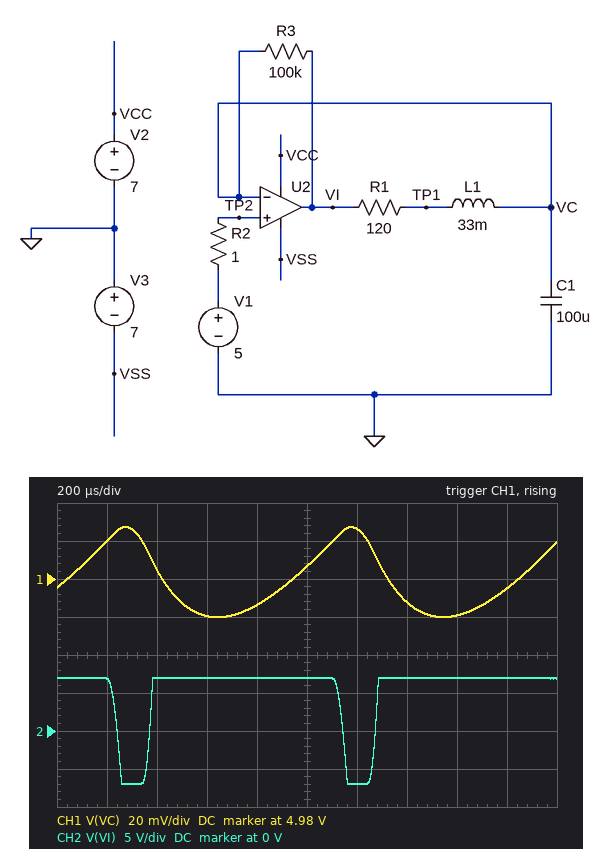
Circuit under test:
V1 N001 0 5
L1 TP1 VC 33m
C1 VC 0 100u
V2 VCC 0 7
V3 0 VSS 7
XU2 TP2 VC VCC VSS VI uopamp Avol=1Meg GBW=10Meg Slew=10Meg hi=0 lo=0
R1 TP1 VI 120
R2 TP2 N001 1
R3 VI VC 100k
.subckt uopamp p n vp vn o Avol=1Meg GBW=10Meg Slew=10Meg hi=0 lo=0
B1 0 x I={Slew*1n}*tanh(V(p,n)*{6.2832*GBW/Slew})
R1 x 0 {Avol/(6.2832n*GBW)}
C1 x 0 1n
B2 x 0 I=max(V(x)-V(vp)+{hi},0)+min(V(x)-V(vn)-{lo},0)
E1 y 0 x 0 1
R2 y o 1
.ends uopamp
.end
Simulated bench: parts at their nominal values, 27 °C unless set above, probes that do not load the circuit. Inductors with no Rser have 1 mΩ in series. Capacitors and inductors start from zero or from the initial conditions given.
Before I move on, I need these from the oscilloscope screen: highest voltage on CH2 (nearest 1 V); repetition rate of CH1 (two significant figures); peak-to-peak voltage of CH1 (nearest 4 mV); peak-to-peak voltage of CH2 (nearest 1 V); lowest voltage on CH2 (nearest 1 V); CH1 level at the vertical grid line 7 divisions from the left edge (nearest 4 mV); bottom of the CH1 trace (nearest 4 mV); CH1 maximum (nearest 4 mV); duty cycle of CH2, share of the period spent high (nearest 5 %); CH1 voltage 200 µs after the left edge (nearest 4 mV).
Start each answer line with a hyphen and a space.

- 7 V
- 1.1 kHz
- 48 mV
- 14 V
- -7 V
- 4.968 V
- 4.960 V
- 5.008 V
- 85 %
- 5.000 V
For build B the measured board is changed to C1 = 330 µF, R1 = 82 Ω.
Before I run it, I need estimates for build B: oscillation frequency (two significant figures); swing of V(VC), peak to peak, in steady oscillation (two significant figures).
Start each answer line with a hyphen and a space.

- 740 Hz
- 32 mV
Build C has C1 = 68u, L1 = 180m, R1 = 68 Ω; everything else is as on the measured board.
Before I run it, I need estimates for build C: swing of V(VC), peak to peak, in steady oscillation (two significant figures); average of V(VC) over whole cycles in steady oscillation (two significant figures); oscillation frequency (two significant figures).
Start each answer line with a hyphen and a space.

- 130 mV
- 4.9 V
- 370 Hz
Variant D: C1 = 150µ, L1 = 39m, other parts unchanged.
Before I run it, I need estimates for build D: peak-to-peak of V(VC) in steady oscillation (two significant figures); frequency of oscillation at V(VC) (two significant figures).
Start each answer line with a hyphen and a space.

- 39 mV
- 920 Hz
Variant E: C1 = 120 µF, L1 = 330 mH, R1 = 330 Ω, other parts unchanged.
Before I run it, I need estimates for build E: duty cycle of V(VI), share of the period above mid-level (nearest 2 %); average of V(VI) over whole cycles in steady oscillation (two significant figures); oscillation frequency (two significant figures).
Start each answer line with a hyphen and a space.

- 84 %
- 4.7 V
- 410 Hz
